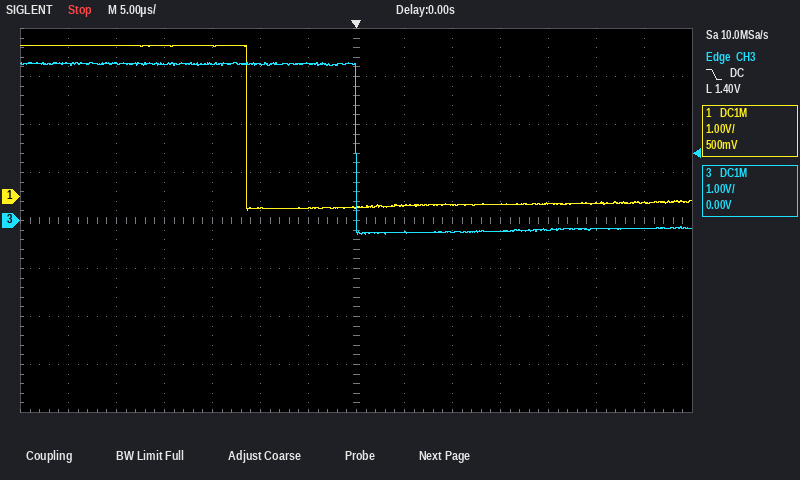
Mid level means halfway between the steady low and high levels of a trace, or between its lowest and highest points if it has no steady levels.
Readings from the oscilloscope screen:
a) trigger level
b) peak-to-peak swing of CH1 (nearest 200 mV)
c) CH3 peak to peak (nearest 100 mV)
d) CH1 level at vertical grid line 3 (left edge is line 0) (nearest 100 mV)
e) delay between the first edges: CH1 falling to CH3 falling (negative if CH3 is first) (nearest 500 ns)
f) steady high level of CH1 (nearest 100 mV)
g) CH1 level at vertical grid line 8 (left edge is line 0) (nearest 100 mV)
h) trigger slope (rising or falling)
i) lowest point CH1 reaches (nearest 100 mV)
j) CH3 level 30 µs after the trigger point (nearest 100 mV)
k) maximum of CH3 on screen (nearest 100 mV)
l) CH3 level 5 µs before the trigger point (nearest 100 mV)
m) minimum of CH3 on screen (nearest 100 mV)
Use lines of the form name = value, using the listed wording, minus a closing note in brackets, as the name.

trigger level = 1.40 V
peak-to-peak swing of CH1 = 3.4 V
CH3 peak to peak = 3.6 V
CH1 level at vertical grid line 3 (left edge is line 0) = 3.1 V
delay between the first edges: CH1 falling to CH3 falling (negative if CH3 is first) = +11.5 µs
steady high level of CH1 = 3.1 V
CH1 level at vertical grid line 8 (left edge is line 0) = -200 mV
trigger slope = falling
lowest point CH1 reaches = -300 mV
CH3 level 30 µs after the trigger point = -200 mV
maximum of CH3 on screen = 3.3 V
CH3 level 5 µs before the trigger point = 3.3 V
minimum of CH3 on screen = -300 mV
